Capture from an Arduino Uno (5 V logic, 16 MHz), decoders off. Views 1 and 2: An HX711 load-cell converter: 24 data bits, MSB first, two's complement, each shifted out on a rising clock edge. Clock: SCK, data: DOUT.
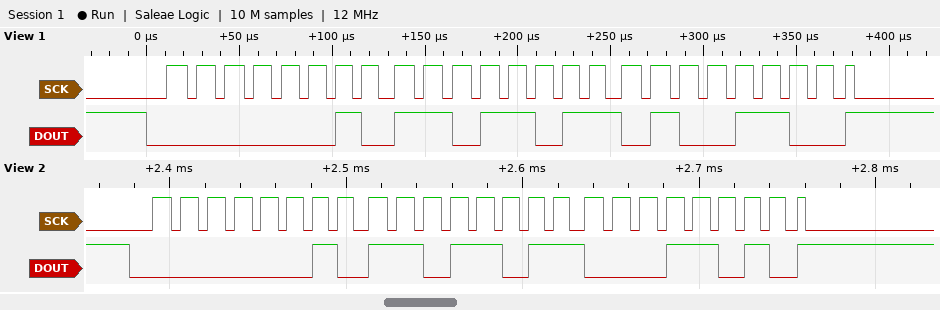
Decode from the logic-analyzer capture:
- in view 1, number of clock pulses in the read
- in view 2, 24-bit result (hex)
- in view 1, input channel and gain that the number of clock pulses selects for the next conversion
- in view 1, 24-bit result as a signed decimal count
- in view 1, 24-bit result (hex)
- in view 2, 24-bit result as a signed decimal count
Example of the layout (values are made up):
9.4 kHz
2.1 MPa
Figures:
25
0x02DB1A
channel A, gain 128
187212
0x02DB4C
187162
